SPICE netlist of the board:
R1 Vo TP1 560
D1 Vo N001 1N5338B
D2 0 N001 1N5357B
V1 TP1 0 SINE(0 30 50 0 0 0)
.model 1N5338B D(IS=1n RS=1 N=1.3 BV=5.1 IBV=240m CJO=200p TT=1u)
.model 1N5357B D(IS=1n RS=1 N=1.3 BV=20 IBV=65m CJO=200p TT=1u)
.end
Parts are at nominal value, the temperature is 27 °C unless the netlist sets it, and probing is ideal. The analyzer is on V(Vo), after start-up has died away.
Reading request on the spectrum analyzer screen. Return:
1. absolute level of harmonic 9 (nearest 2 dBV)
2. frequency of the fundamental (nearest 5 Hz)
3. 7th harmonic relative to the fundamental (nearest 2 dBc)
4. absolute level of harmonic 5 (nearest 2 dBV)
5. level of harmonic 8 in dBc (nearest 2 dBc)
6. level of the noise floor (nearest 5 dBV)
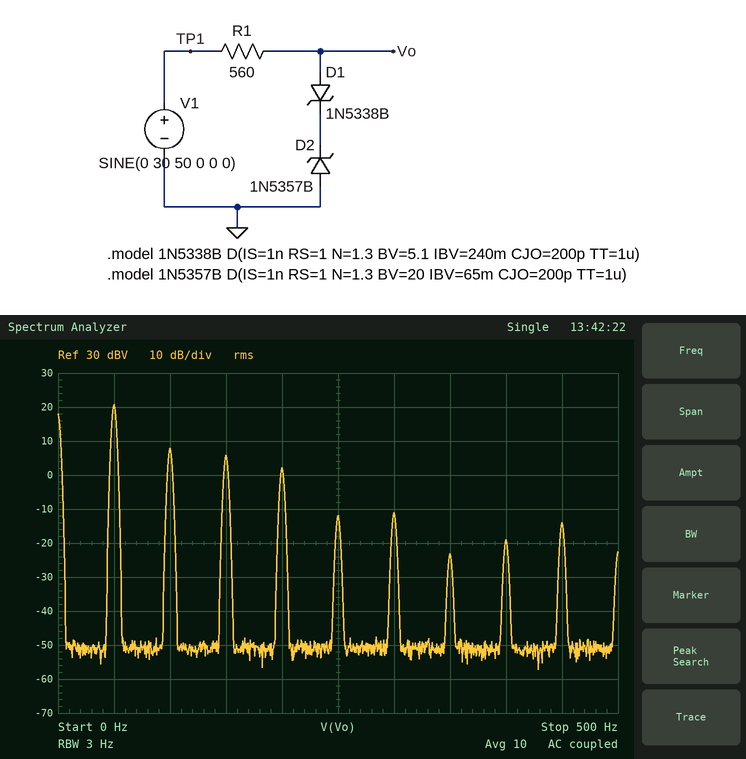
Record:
-14 dBV
50 Hz
-44 dBc
-12 dBV
-40 dBc
-50 dBV
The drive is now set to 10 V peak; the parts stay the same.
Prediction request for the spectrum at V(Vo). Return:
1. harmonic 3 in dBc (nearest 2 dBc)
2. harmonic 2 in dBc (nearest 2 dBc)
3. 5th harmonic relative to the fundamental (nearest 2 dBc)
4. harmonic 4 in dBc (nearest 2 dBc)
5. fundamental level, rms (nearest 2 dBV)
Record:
-22 dBc
-16 dBc
-40 dBc
-34 dBc
16 dBV
